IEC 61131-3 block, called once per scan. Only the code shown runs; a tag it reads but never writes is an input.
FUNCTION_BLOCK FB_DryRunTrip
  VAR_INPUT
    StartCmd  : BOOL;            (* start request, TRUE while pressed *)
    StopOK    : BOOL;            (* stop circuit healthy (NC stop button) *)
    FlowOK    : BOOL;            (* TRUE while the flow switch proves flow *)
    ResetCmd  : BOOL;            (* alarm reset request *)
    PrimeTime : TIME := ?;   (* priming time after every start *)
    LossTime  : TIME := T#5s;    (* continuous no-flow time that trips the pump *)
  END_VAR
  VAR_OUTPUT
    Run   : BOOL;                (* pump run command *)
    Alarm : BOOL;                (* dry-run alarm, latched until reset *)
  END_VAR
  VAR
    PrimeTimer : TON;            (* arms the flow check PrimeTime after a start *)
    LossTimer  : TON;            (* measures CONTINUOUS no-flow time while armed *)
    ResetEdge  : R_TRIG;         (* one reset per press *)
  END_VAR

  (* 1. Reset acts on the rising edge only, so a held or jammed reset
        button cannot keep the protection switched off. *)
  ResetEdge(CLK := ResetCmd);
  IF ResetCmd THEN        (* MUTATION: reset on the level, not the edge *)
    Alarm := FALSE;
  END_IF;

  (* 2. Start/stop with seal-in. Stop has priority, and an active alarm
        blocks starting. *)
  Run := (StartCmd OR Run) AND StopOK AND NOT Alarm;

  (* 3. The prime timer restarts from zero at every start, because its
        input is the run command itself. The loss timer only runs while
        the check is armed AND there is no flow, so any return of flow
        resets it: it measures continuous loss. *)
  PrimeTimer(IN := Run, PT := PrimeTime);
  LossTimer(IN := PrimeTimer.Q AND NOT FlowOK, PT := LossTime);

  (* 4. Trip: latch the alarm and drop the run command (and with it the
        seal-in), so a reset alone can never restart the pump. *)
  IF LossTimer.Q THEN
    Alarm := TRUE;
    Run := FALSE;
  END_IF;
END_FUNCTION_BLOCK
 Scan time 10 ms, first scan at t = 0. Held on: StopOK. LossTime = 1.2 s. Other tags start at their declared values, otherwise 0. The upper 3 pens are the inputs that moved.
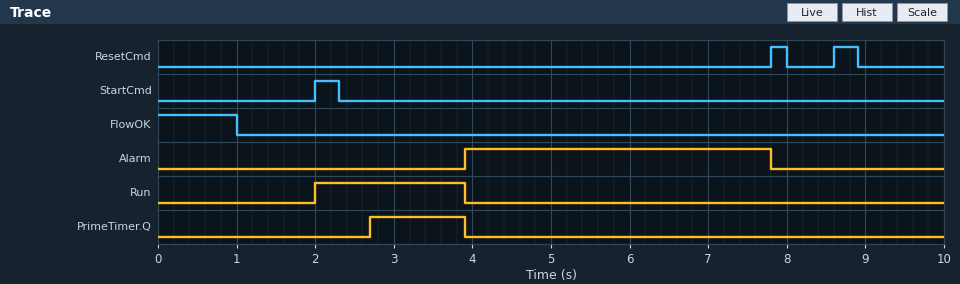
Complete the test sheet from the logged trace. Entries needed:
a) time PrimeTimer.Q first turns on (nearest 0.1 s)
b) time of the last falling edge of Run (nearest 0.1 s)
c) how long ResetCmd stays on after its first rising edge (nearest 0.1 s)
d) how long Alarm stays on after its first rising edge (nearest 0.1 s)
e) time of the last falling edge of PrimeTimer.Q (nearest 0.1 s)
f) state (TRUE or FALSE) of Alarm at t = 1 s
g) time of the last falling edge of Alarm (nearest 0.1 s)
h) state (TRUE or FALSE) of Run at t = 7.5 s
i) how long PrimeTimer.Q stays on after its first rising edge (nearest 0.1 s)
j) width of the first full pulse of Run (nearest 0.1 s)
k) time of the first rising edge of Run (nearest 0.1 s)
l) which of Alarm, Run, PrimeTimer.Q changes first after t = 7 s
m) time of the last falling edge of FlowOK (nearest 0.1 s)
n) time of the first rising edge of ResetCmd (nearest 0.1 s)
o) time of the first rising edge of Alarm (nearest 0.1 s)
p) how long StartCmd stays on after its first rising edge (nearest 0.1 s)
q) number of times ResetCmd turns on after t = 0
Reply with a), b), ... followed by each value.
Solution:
a) 2.7 s
b) 3.9 s
c) 0.2 s
d) 3.9 s
e) 3.9 s
f) FALSE
g) 7.8 s
h) FALSE
i) 1.2 s
j) 1.9 s
k) 2.0 s
l) Alarm
m) 1.0 s
n) 7.8 s
o) 3.9 s
p) 0.3 s
q) 2
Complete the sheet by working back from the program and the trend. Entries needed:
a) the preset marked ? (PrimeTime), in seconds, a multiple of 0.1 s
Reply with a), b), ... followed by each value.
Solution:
a) 0.7 s
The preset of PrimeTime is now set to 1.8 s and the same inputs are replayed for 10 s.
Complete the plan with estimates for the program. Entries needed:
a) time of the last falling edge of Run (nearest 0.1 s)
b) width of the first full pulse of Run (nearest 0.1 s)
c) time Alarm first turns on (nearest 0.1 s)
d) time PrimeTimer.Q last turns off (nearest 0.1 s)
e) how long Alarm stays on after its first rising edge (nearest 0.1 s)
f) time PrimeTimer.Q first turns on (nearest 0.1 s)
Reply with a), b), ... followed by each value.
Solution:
a) 5.0 s
b) 3.0 s
c) 5.0 s
d) 5.0 s
e) 2.8 s
f) 3.8 s
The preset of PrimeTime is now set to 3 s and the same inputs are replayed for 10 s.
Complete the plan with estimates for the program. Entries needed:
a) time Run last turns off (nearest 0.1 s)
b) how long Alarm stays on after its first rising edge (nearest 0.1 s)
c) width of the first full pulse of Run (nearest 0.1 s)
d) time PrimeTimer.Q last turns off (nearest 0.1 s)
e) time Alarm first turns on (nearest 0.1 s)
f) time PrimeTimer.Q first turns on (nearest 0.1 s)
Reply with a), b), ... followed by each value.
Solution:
a) 6.2 s
b) 1.6 s
c) 4.2 s
d) 6.2 s
e) 6.2 s
f) 5.0 s
